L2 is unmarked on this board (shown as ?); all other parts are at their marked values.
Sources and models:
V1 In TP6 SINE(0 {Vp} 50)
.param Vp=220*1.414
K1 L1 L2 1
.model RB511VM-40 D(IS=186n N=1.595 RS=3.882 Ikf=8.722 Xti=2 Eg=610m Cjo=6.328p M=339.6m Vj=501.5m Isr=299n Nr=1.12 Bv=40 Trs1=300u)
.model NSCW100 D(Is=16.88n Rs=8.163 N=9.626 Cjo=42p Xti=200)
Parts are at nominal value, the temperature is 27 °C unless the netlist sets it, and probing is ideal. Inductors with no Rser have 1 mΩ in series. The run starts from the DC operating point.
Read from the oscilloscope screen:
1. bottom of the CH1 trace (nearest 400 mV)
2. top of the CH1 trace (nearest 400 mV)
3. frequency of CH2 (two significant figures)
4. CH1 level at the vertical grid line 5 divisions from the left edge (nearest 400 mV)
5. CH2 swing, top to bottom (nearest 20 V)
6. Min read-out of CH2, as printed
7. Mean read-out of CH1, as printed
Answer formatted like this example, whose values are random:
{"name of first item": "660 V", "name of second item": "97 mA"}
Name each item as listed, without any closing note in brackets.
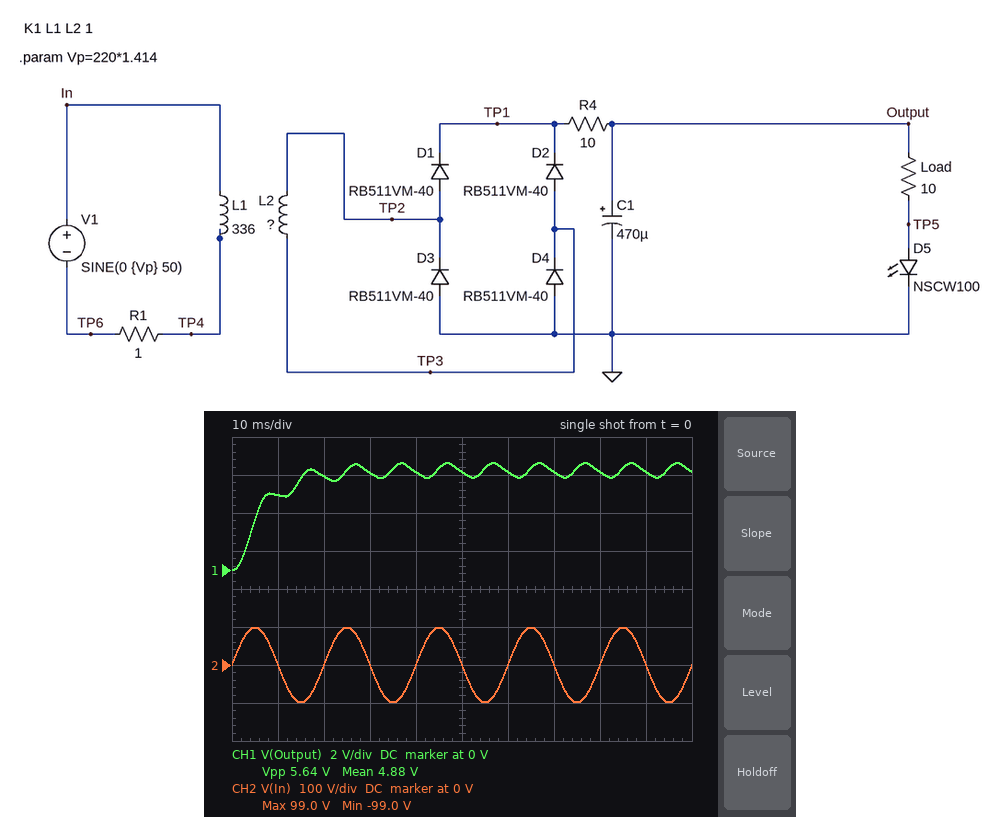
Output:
{"bottom of the CH1 trace": "0 V", "top of the CH1 trace": "5.6 V", "frequency of CH2": "50 Hz", "CH1 level at the vertical grid line 5 divisions from the left edge": "5.2 V", "CH2 swing, top to bottom": "200 V", "Min read-out of CH2, as printed": "-99.0 V", "Mean read-out of CH1, as printed": "4.88 V"}
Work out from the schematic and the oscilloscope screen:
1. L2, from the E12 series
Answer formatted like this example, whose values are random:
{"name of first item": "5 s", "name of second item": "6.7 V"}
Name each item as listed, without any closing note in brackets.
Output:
{"L2, from the E12 series": "330 mH"}
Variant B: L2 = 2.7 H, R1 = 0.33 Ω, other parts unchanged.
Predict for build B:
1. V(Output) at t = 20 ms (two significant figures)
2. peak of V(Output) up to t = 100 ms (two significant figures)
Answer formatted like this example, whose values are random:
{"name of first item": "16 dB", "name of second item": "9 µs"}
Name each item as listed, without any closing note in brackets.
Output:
{"V(Output) at t = 20 ms": "11 V", "peak of V(Output) up to t = 100 ms": "13 V"}
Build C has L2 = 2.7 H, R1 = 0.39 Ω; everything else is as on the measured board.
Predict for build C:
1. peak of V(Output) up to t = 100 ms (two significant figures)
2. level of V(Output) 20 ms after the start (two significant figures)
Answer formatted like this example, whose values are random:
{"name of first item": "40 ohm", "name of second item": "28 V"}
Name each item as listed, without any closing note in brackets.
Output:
{"peak of V(Output) up to t = 100 ms": "13 V", "level of V(Output) 20 ms after the start": "11 V"}
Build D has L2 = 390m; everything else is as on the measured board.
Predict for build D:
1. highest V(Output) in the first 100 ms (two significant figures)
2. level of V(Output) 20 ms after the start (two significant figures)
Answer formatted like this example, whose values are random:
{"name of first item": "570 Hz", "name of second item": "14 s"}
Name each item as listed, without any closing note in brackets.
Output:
{"highest V(Output) in the first 100 ms": "6.0 V", "level of V(Output) 20 ms after the start": "5.2 V"}
